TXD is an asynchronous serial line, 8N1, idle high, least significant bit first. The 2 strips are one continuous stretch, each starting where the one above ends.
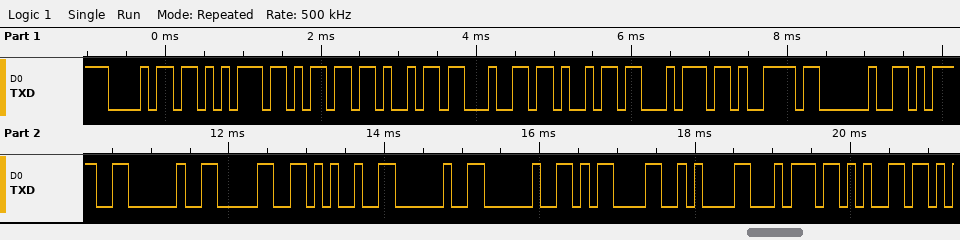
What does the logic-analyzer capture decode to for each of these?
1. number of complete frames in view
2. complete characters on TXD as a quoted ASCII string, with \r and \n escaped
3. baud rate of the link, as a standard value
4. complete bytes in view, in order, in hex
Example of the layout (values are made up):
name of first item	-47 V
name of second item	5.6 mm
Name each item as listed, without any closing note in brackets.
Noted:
number of complete frames in view	19
complete characters on TXD as a quoted ASCII string, with \r and \n escaped	"humidity = 0%  \r\nte"
baud rate of the link, as a standard value	9600 baud
complete bytes in view, in order, in hex	0x68 0x75 0x6D 0x69 0x64 0x69 0x74 0x79 0x20 0x3D 0x20 0x30 0x25 0x20 0x20 0x0D 0x0A 0x74 0x65
